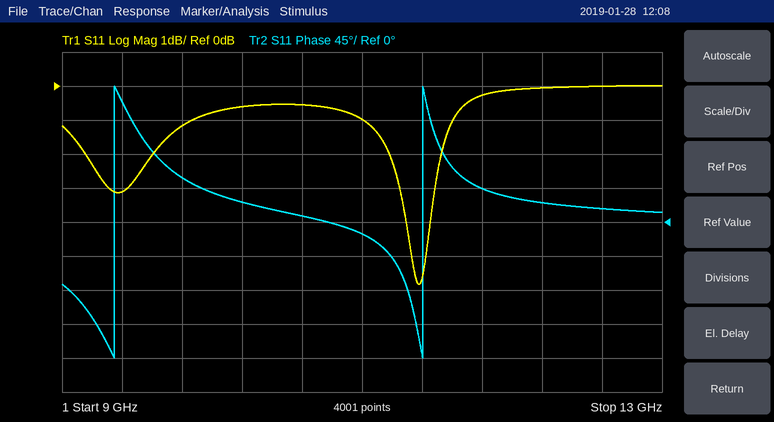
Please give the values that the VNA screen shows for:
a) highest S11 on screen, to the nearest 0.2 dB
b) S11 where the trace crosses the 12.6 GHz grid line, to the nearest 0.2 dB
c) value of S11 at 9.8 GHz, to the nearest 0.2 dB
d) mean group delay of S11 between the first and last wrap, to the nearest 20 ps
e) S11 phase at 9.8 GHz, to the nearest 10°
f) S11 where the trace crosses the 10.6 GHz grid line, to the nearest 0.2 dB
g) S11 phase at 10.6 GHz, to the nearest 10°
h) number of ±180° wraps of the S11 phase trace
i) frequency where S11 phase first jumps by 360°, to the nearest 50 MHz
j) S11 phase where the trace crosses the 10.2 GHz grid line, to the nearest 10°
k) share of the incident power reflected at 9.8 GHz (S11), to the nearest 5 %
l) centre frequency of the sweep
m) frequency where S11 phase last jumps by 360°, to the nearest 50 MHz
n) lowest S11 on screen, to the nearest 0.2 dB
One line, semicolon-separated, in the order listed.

0.0 dB; 0.0 dB; -1.2 dB; 480 ps; 60°; -0.6 dB; 10°; 2; 9.35 GHz; 30°; 75 %; 11 GHz; 11.40 GHz; -5.8 dB
